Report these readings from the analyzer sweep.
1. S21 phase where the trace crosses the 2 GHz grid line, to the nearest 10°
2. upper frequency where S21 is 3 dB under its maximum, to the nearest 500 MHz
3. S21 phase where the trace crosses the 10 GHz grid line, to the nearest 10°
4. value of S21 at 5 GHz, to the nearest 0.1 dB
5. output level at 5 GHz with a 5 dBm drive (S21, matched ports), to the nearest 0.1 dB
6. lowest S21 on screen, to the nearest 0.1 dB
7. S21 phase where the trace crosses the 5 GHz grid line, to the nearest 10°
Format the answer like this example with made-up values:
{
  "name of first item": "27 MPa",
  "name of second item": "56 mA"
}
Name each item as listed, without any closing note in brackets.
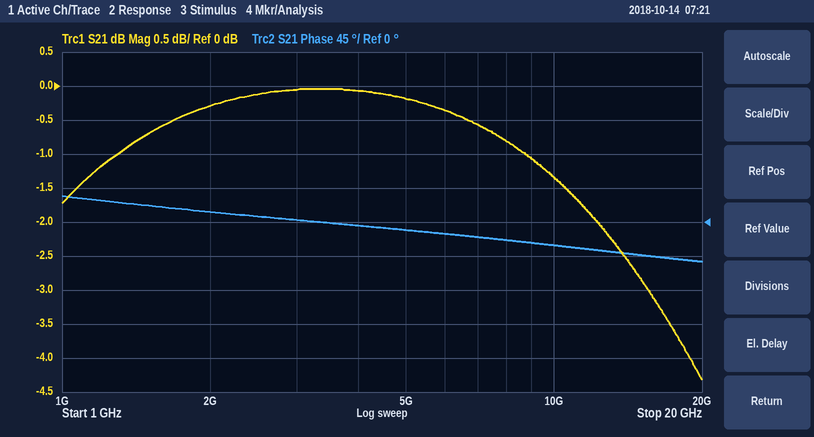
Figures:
{
  "S21 phase where the trace crosses the 2 GHz grid line, to the nearest 10°": "10°",
  "upper frequency where S21 is 3 dB under its maximum, to the nearest 500 MHz": "15.5 GHz",
  "S21 phase where the trace crosses the 10 GHz grid line, to the nearest 10°": "-30°",
  "value of S21 at 5 GHz, to the nearest 0.1 dB": "-0.2 dB",
  "output level at 5 GHz with a 5 dBm drive (S21, matched ports), to the nearest 0.1 dB": "4.8 dBm",
  "lowest S21 on screen, to the nearest 0.1 dB": "-4.3 dB",
  "S21 phase where the trace crosses the 5 GHz grid line, to the nearest 10°": "-10°"
}
